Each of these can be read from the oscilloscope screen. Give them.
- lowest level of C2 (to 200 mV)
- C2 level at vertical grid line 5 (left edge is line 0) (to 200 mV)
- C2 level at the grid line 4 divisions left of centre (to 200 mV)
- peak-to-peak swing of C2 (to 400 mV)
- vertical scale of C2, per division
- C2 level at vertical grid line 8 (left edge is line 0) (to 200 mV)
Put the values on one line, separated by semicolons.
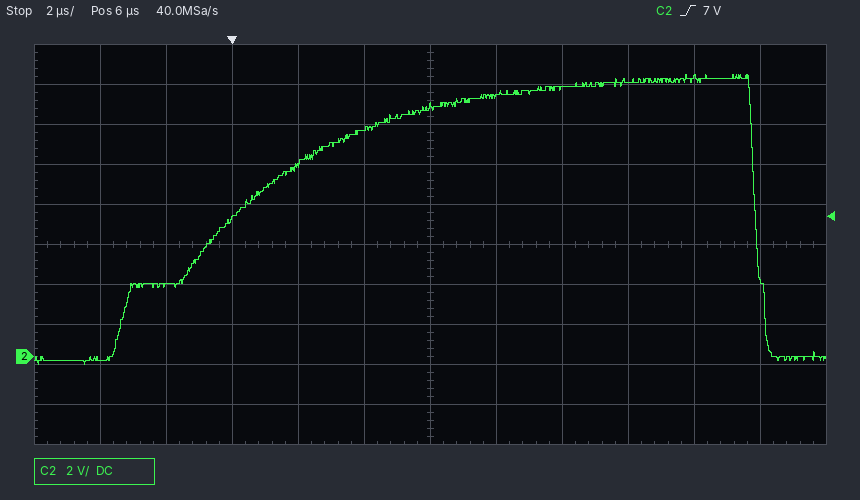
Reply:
-400 mV; 11.4 V; 3.6 V; 14.4 V; 2 V; 13.4 V
